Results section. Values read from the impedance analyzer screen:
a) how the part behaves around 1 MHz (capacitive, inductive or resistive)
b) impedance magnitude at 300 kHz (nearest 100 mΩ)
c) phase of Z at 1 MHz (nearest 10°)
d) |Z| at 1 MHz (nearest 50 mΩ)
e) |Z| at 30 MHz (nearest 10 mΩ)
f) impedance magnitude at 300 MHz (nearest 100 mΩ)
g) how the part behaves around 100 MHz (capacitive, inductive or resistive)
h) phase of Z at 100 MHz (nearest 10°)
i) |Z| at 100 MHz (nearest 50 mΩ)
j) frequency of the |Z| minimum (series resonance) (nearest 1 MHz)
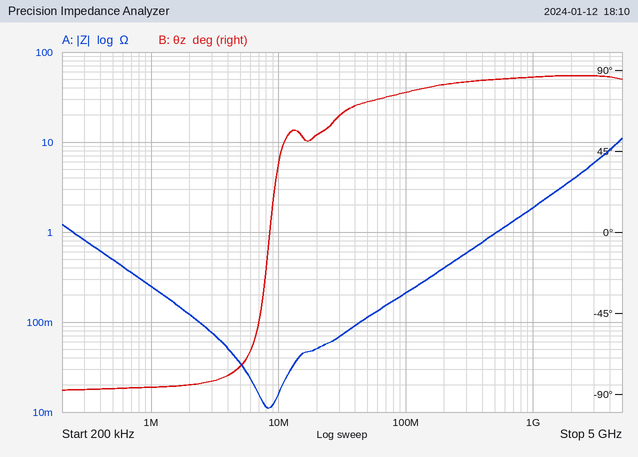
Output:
capacitive
800 mΩ
-90°
250 mΩ
70 mΩ
600 mΩ
inductive
80°
200 mΩ
8 MHz
